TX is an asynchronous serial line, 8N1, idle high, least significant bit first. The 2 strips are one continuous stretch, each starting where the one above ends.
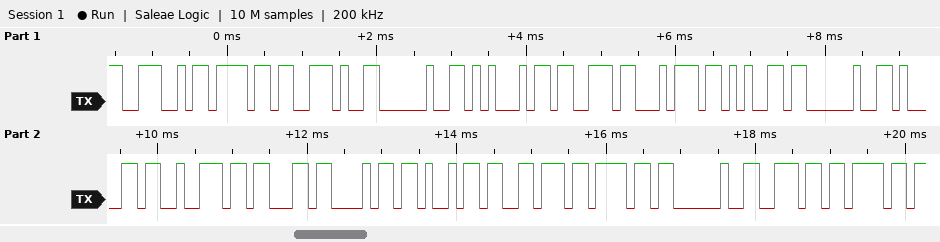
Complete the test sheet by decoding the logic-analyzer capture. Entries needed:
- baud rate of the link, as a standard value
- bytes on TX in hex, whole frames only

9600 baud
0x4E 0x6F 0x2E 0x20 0x45 0x73 0x74 0x65 0x20 0x61 0x72 0x63 0x68 0x69 0x76 0x6F 0x20 0x6E 0x6F
